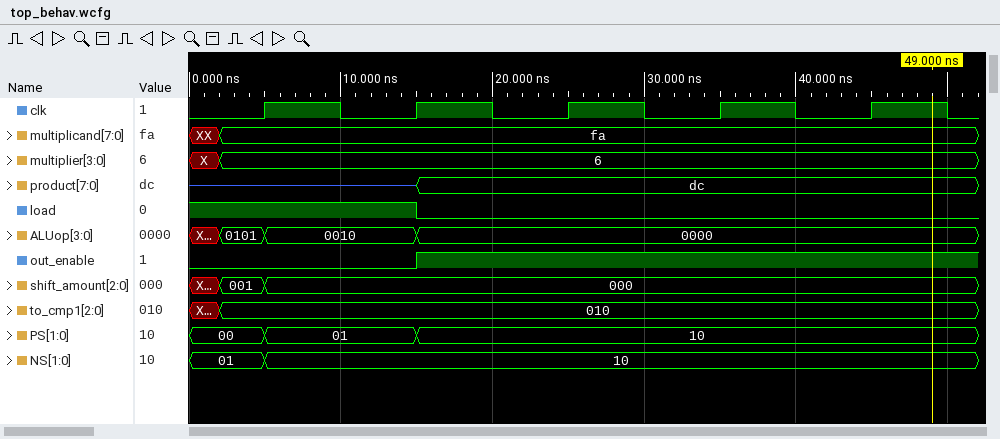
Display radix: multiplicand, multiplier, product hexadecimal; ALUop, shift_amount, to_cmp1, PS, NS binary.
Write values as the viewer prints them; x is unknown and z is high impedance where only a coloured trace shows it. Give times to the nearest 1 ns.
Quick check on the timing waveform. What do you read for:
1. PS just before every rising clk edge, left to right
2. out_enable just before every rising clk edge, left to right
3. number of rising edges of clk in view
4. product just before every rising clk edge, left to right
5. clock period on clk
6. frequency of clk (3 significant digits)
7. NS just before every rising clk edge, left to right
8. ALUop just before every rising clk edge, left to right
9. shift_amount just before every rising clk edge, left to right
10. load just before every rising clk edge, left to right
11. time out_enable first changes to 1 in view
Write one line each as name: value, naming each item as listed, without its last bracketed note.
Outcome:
PS just before every rising clk edge, left to right: 00, 01, 10, 10, 10
out_enable just before every rising clk edge, left to right: 0 0 1 1 1
number of rising edges of clk in view: 5
product just before every rising clk edge, left to right: z, z, dc, dc, dc
clock period on clk: 10 ns
frequency of clk: 100 MHz
NS just before every rising clk edge, left to right: 01, 10, 10, 10, 10
ALUop just before every rising clk edge, left to right: 0101, 0010, 0000, 0000, 0000
shift_amount just before every rising clk edge, left to right: 001, 000, 000, 000, 000
load just before every rising clk edge, left to right: 1 1 0 0 0
time out_enable first changes to 1 in view: 15 ns
